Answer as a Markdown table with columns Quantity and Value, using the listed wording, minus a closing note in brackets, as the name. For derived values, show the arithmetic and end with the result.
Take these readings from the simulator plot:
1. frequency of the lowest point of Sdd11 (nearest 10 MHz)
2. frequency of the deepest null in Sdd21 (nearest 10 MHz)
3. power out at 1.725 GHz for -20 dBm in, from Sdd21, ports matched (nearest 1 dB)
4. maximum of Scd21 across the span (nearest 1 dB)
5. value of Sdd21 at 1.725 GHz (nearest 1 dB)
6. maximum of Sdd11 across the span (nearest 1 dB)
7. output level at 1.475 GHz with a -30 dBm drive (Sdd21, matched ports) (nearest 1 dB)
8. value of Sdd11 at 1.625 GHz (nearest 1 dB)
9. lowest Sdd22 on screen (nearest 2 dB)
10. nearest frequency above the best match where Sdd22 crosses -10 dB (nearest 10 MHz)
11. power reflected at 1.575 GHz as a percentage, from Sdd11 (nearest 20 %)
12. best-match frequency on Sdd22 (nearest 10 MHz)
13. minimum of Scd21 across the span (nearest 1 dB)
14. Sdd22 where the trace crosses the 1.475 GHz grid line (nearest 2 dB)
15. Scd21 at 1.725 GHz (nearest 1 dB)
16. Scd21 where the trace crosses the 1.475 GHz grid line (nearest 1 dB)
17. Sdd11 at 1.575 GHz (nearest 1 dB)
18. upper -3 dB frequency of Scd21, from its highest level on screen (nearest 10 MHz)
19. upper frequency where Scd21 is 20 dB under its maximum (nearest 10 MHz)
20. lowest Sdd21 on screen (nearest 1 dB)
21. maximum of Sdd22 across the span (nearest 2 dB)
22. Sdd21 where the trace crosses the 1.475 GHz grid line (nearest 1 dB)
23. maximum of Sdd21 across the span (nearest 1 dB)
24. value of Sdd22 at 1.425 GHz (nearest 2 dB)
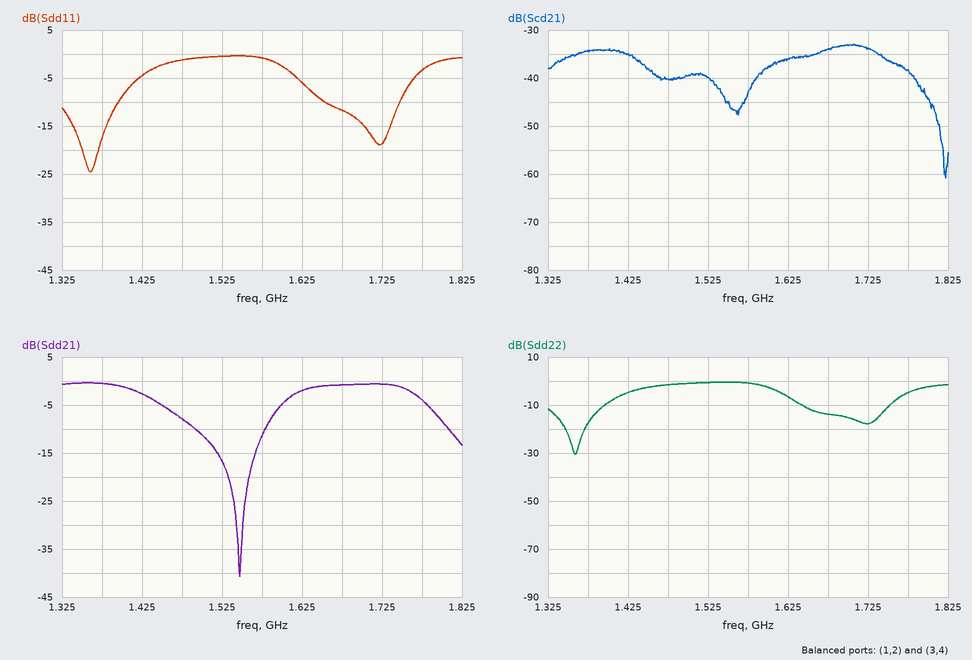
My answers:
| Quantity | Value |
|---|---|
| frequency of the lowest point of Sdd11 | 1.36 GHz |
| frequency of the deepest null in Sdd21 | 1.55 GHz |
| power out at 1.725 GHz for -20 dBm in, from Sdd21, ports matched | -20 dBm + (-1 dB) = -21 dBm |
| maximum of Scd21 across the span | -33 dB |
| value of Sdd21 at 1.725 GHz | -1 dB |
| maximum of Sdd11 across the span | 0 dB |
| output level at 1.475 GHz with a -30 dBm drive (Sdd21, matched ports) | -30 dBm + (-8 dB) = -38 dBm |
| value of Sdd11 at 1.625 GHz | -6 dB |
| lowest Sdd22 on screen | -30 dB |
| nearest frequency above the best match where Sdd22 crosses -10 dB | 1.40 GHz |
| power reflected at 1.575 GHz as a percentage, from Sdd11 | 10^(-1/10) ≈ 79.4 %, so 80 % to the nearest 20 % |
| best-match frequency on Sdd22 | 1.36 GHz |
| minimum of Scd21 across the span | -61 dB |
| Sdd22 where the trace crosses the 1.475 GHz grid line | -2 dB |
| Scd21 at 1.725 GHz | -34 dB |
| Scd21 where the trace crosses the 1.475 GHz grid line | -40 dB |
| Sdd11 at 1.575 GHz | -1 dB |
| upper -3 dB frequency of Scd21, from its highest level on screen | 1.75 GHz |
| upper frequency where Scd21 is 20 dB under its maximum | 1.82 GHz |
| lowest Sdd21 on screen | -41 dB |
| maximum of Sdd22 across the span | 0 dB |
| Sdd21 where the trace crosses the 1.475 GHz grid line | -8 dB |
| maximum of Sdd21 across the span | 0 dB |
| value of Sdd22 at 1.425 GHz | -4 dB |
